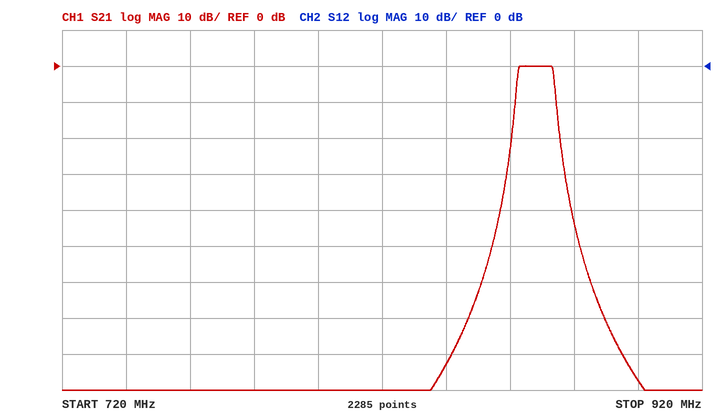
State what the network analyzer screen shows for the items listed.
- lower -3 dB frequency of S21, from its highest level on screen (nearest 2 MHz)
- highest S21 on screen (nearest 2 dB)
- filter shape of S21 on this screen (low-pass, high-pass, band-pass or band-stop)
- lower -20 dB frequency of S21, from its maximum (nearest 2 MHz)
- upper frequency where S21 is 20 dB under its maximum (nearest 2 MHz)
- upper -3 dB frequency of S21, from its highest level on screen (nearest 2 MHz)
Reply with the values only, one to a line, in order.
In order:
862 MHz
0 dB
band-pass
860 MHz
876 MHz
874 MHz
